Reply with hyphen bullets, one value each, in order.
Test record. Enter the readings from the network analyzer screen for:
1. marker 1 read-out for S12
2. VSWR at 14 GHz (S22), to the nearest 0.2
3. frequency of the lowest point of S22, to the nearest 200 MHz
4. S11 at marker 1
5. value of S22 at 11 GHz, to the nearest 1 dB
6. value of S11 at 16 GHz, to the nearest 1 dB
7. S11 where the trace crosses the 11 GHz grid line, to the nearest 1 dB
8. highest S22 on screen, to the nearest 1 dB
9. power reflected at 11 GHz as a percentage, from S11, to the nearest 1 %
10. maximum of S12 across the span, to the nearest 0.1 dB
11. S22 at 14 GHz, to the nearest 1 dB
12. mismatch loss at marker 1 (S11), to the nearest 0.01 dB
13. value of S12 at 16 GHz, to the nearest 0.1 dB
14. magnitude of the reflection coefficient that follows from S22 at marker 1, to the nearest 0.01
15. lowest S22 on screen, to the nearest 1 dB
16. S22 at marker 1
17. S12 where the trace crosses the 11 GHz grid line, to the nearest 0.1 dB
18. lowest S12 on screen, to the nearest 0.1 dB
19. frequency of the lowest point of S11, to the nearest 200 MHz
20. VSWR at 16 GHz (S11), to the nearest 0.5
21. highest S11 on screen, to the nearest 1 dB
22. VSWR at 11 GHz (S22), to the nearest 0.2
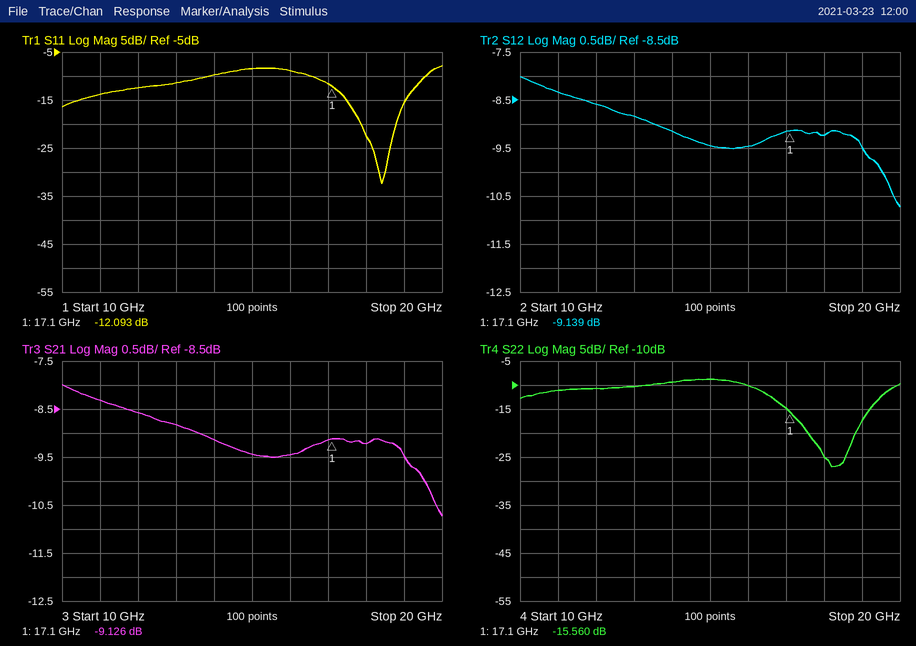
- -9.139 dB
- 2.0
- 18.2 GHz
- -12.093 dB
- -11 dB
- -9 dB
- -14 dB
- -9 dB
- 4 %
- -8.0 dB
- -9 dB
- 0.28 dB
- -9.5 dB
- 0.17
- -27 dB
- -15.560 dB
- -8.3 dB
- -10.7 dB
- 18.4 GHz
- 2.0
- -8 dB
- 1.8
